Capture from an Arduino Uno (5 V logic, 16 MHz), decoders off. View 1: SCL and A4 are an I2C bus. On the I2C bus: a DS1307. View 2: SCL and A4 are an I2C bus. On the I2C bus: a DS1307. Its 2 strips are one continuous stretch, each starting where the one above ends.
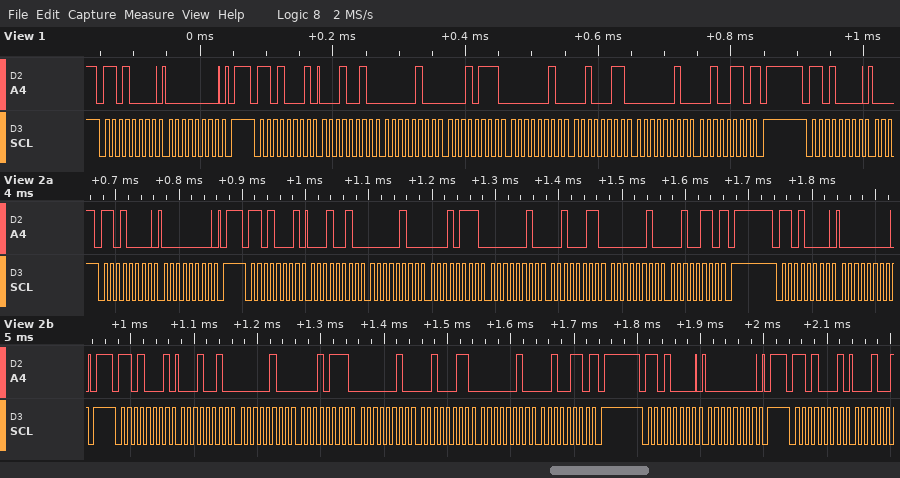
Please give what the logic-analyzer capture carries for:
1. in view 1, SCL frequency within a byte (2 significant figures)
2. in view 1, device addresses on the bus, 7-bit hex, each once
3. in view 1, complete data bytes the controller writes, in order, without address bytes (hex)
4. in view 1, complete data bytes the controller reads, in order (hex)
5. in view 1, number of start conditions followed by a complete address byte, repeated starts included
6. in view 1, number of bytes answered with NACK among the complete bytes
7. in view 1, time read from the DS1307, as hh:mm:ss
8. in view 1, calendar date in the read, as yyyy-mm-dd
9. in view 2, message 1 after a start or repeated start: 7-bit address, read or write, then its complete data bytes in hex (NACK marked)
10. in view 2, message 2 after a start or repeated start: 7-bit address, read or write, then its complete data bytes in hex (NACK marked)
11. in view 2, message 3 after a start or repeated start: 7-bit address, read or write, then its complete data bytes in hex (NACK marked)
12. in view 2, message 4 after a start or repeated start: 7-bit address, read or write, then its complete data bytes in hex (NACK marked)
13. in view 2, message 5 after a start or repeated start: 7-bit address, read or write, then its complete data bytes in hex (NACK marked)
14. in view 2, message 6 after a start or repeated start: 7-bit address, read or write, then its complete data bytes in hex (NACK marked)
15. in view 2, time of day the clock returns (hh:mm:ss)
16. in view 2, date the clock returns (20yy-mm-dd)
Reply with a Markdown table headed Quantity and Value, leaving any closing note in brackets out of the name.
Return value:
| Quantity | Value |
|---|---|
| in view 1, SCL frequency within a byte | 100 kHz |
| in view 1, device addresses on the bus, 7-bit hex, each once | 0x68 |
| in view 1, complete data bytes the controller writes, in order, without address bytes | 00 |
| in view 1, complete data bytes the controller reads, in order | 12 04 17 02 23 02 26 |
| in view 1, number of start conditions followed by a complete address byte, repeated starts included | 3 |
| in view 1, number of bytes answered with NACK among the complete bytes | 1 |
| in view 1, time read from the DS1307, as hh:mm:ss | 17:04:12 |
| in view 1, calendar date in the read, as yyyy-mm-dd | 2026-02-23 |
| in view 2, message 1 after a start or repeated start: 7-bit address, read or write, then its complete data bytes in hex | 0x68 write: 00 |
| in view 2, message 2 after a start or repeated start: 7-bit address, read or write, then its complete data bytes in hex | 0x68 read: 12 04 17 02 23 02 26 NACK |
| in view 2, message 3 after a start or repeated start: 7-bit address, read or write, then its complete data bytes in hex | 0x68 write: 00 |
| in view 2, message 4 after a start or repeated start: 7-bit address, read or write, then its complete data bytes in hex | 0x68 read: 12 04 17 02 23 02 26 NACK |
| in view 2, message 5 after a start or repeated start: 7-bit address, read or write, then its complete data bytes in hex | 0x68 write: 00 |
| in view 2, message 6 after a start or repeated start: 7-bit address, read or write, then its complete data bytes in hex | 0x68 read |
| in view 2, time of day the clock returns | 17:04:12 |
| in view 2, date the clock returns | 2026-02-23 |
